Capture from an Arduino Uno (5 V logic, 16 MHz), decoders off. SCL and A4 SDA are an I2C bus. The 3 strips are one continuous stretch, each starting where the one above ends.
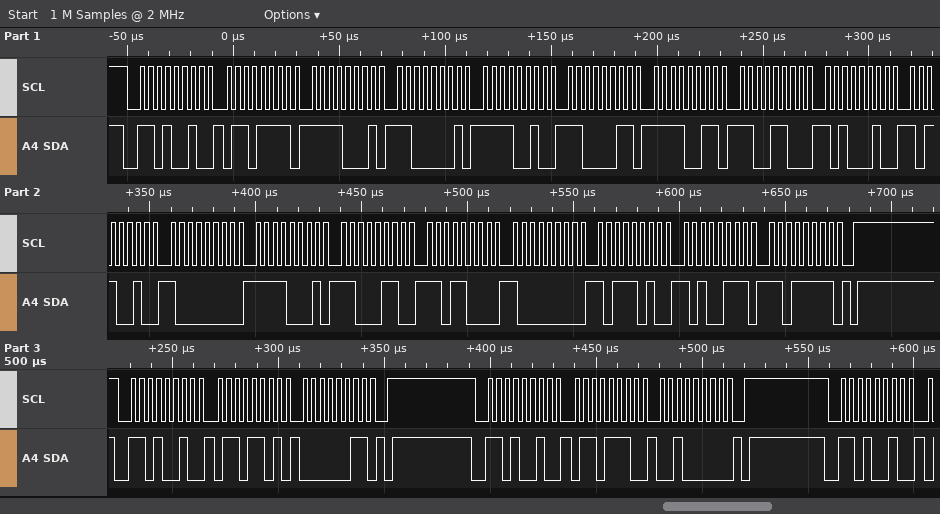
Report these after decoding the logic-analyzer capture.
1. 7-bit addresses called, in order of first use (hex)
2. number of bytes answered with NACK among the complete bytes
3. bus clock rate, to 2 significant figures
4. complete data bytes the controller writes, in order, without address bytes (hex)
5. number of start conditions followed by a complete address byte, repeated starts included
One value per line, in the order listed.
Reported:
0x69
0
250 kHz
6F F1 C1 F2 C3 F3 CC A2 B2 80 F1 C6 D8 80 BA A7 DF 6D 03 6E 20
4
